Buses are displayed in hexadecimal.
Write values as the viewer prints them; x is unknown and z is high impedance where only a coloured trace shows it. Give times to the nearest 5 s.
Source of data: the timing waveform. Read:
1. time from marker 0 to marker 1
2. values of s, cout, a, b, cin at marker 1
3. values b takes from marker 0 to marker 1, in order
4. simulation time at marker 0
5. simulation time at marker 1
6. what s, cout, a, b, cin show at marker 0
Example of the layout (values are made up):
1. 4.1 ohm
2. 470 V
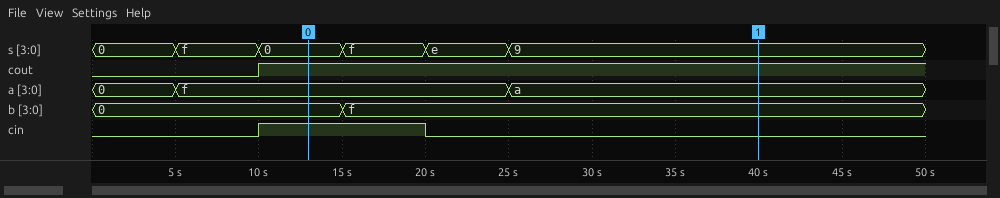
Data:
1. 25 s
2. s=9, cout=1, a=a, b=f, cin=0
3. 0, f
4. 15 s
5. 40 s
6. s=0, cout=1, a=f, b=0, cin=1
